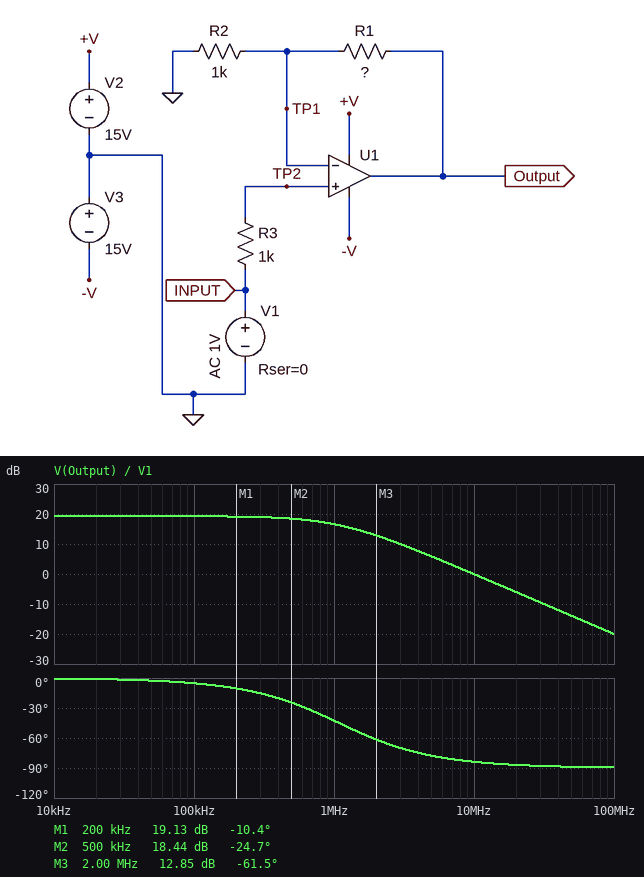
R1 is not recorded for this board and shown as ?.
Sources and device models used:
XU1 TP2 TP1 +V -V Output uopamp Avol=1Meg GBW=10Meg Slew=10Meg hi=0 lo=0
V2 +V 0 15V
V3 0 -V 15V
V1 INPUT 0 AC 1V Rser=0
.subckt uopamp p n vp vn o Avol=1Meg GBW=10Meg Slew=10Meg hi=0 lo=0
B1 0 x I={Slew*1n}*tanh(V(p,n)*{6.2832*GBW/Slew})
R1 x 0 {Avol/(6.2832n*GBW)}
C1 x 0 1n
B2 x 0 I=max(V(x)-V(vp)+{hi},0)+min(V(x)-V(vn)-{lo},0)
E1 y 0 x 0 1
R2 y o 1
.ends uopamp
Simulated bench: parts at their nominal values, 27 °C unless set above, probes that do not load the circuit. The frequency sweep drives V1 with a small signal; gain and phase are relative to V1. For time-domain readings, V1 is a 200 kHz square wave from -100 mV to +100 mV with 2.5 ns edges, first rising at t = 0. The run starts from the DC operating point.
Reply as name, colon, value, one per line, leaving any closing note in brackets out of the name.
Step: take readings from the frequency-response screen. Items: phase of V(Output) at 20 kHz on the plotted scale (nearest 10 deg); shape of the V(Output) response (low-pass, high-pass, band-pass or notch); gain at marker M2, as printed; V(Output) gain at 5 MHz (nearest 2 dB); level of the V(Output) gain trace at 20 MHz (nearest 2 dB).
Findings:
phase of V(Output) at 20 kHz on the plotted scale: 0 deg
shape of the V(Output) response: low-pass
gain at marker M2, as printed: 18.44 dB
V(Output) gain at 5 MHz: 6 dB
level of the V(Output) gain trace at 20 MHz: -6 dB
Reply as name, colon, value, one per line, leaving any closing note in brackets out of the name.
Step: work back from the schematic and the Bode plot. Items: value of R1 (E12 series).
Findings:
value of R1: 8.2 kΩ
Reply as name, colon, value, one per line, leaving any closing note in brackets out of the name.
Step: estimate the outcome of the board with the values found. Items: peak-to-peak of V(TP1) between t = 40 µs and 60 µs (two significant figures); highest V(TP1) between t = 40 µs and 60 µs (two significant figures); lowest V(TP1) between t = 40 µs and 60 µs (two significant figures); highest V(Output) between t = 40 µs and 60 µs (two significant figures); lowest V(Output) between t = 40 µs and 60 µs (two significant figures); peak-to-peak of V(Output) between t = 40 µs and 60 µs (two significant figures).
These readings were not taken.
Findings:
peak-to-peak of V(TP1) between t = 40 µs and 60 µs: 200 mV
highest V(TP1) between t = 40 µs and 60 µs: 100 mV
lowest V(TP1) between t = 40 µs and 60 µs: -100 mV
highest V(Output) between t = 40 µs and 60 µs: 920 mV
lowest V(Output) between t = 40 µs and 60 µs: -920 mV
peak-to-peak of V(Output) between t = 40 µs and 60 µs: 1.8 V
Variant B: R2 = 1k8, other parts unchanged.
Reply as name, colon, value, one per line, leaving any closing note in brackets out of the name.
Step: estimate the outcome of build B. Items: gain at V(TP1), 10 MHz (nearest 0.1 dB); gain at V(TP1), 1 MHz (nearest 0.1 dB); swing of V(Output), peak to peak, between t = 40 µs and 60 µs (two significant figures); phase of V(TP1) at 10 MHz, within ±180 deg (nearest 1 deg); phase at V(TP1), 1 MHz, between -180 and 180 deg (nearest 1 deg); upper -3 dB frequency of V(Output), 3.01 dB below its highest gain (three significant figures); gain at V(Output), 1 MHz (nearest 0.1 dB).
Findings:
gain at V(TP1), 10 MHz: -15.0 dB
gain at V(TP1), 1 MHz: -1.2 dB
swing of V(Output), peak to peak, between t = 40 µs and 60 µs: 1.1 V
phase of V(TP1) at 10 MHz, within ±180 deg: -80 deg
phase at V(TP1), 1 MHz, between -180 and 180 deg: -29 deg
upper -3 dB frequency of V(Output), 3.01 dB below its highest gain: 1.80 MHz
gain at V(Output), 1 MHz: 13.7 dB
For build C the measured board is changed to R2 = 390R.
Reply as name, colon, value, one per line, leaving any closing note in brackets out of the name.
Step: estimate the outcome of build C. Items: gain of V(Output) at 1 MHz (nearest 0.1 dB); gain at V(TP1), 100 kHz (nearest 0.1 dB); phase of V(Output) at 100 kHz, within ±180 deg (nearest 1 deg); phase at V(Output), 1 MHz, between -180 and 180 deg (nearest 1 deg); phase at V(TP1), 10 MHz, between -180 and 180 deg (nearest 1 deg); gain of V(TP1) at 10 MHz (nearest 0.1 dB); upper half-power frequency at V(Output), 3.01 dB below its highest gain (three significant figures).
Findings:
gain of V(Output) at 1 MHz: 19.2 dB
gain at V(TP1), 100 kHz: -0.2 dB
phase of V(Output) at 100 kHz, within ±180 deg: -12 deg
phase at V(Output), 1 MHz, between -180 and 180 deg: -66 deg
phase at V(TP1), 10 MHz, between -180 and 180 deg: -87 deg
gain of V(TP1) at 10 MHz: -26.9 dB
upper half-power frequency at V(Output), 3.01 dB below its highest gain: 454 kHz
